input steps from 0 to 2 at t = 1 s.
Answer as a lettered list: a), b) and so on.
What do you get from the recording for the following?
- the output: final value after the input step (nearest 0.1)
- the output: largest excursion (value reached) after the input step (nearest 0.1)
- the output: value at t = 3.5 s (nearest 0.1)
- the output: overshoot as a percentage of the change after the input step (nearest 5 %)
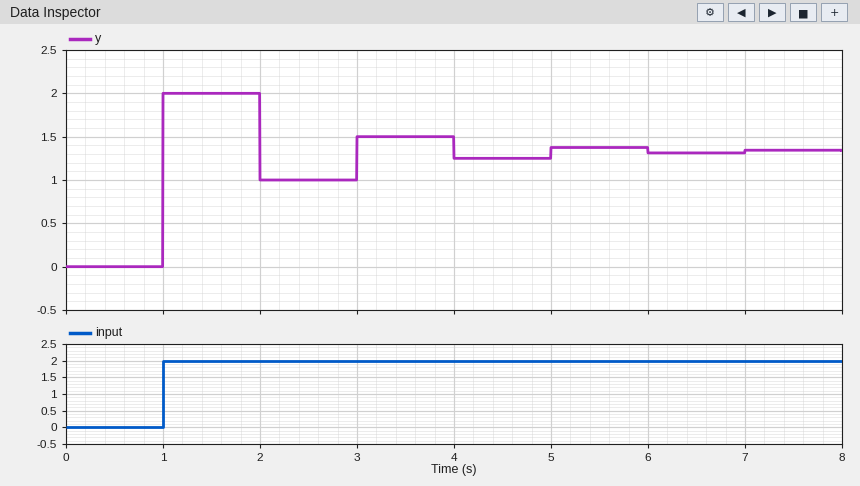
a) 1.3
b) 2.0
c) 1.5
d) 50 %
